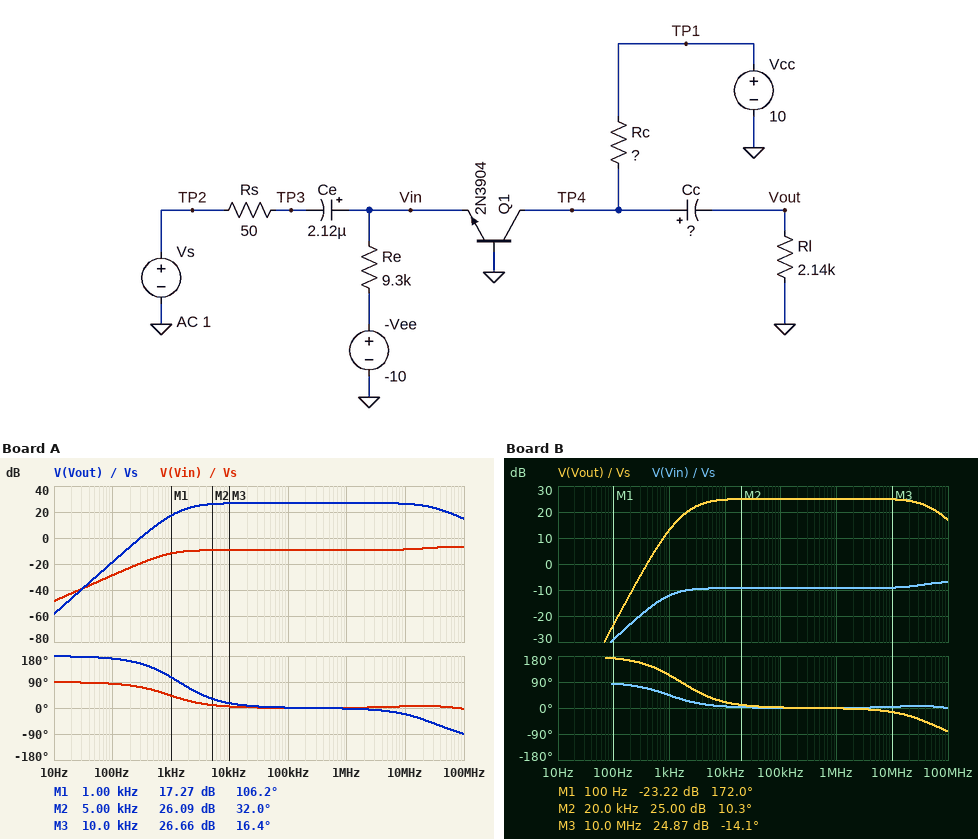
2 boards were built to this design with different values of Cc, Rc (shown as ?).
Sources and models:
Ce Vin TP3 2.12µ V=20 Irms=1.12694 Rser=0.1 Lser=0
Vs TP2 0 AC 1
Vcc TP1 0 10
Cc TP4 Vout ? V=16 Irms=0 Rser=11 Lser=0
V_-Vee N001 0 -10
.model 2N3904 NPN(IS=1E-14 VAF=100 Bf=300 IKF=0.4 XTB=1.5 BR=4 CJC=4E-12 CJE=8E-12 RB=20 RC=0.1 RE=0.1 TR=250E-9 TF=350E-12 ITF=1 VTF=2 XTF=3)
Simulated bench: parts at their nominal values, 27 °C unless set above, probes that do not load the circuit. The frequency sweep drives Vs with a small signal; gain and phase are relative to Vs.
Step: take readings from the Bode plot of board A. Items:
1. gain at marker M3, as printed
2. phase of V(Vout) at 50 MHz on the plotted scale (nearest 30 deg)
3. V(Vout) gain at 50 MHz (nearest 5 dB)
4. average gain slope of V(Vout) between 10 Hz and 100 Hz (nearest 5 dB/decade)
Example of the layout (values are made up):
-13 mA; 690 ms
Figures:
26.66 dB; -60 deg; 20 dB; 40 dB/decade
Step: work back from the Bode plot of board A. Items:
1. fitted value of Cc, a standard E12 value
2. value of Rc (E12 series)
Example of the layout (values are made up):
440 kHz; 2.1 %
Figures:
8.2 nF; 8.2 kΩ
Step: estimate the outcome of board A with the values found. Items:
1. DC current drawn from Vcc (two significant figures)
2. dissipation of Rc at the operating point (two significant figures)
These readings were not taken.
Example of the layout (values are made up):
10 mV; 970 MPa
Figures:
1.0 mA; 8.2 mW
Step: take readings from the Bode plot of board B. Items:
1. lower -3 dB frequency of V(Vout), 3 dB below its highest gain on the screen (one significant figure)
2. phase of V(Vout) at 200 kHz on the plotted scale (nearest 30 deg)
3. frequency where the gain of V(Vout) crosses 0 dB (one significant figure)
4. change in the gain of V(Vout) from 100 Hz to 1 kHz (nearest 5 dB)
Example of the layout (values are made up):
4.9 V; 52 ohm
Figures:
3 kHz; 0 deg; 400 Hz; 35 dB
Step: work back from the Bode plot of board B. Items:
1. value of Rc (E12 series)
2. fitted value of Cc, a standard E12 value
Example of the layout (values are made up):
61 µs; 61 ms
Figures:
3.9 kΩ; 10 nF
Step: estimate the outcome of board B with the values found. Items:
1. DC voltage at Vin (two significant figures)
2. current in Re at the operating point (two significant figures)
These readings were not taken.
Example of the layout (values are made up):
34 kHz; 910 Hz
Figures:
-650 mV; 1.0 mA
